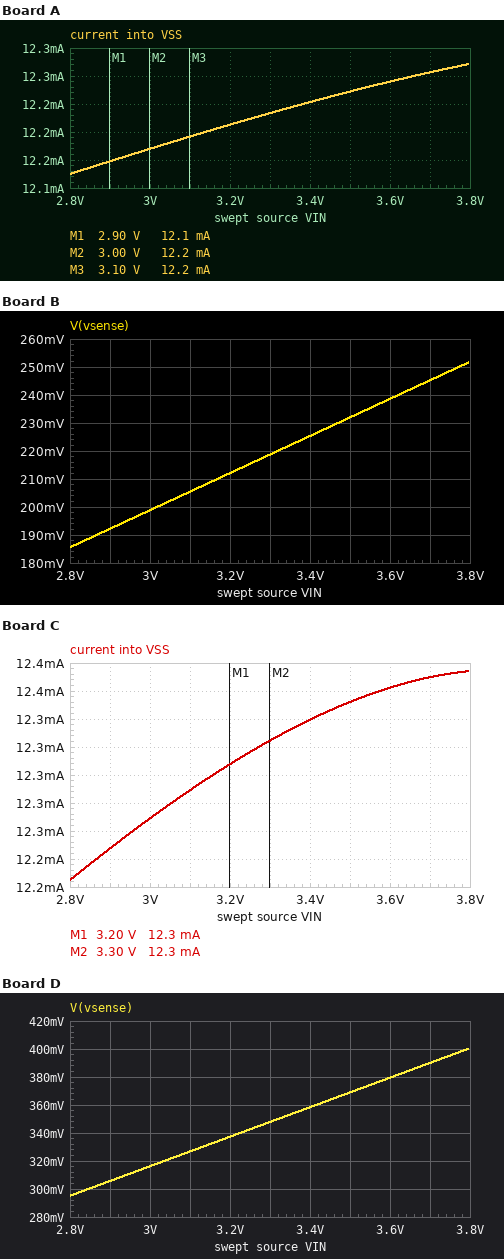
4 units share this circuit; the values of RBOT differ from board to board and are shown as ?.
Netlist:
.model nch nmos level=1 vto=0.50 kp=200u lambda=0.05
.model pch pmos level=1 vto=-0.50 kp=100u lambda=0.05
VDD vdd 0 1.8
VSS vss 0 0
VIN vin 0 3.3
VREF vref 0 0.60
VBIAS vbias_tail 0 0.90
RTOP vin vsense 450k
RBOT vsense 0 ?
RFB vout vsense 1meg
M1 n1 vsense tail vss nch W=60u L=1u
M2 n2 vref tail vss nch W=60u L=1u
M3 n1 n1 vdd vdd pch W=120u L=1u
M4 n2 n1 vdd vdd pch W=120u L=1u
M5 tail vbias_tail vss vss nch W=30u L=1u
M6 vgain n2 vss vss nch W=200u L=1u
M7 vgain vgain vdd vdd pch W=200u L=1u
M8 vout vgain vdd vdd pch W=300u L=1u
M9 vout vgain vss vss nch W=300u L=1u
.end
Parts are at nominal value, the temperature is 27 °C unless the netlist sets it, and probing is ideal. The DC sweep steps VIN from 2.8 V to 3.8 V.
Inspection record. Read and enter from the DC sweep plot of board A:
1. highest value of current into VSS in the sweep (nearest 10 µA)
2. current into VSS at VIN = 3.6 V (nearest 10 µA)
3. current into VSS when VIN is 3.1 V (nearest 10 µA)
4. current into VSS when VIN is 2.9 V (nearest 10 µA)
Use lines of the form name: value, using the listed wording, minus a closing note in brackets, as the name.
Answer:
highest value of current into VSS in the sweep: 12.32 mA
current into VSS at VIN = 3.6 V: 12.29 mA
current into VSS when VIN is 3.1 V: 12.19 mA
current into VSS when VIN is 2.9 V: 12.15 mA
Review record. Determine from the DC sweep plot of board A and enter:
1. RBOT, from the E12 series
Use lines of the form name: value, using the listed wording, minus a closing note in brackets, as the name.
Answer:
RBOT, from the E12 series: 150 kΩ
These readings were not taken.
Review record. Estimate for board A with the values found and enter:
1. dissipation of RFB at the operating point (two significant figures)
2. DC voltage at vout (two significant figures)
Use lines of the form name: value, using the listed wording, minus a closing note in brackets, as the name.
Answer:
dissipation of RFB at the operating point: 770 nW
DC voltage at vout: 1.8 V
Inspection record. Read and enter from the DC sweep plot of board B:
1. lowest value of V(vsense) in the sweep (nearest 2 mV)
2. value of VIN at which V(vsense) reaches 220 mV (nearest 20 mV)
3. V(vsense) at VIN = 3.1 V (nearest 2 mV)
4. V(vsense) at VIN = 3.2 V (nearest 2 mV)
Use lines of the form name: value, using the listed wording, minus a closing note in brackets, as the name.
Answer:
lowest value of V(vsense) in the sweep: 186 mV
value of VIN at which V(vsense) reaches 220 mV: 3.32 V
V(vsense) at VIN = 3.1 V: 206 mV
V(vsense) at VIN = 3.2 V: 212 mV
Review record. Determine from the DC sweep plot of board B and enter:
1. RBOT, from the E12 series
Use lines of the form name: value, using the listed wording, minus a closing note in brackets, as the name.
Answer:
RBOT, from the E12 series: 33 kΩ
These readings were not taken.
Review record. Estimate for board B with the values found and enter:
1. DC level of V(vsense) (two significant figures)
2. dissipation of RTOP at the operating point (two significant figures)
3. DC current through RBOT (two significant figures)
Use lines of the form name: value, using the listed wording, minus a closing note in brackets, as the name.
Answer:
DC level of V(vsense): 220 mV
dissipation of RTOP at the operating point: 21 µW
DC current through RBOT: 6.6 µA
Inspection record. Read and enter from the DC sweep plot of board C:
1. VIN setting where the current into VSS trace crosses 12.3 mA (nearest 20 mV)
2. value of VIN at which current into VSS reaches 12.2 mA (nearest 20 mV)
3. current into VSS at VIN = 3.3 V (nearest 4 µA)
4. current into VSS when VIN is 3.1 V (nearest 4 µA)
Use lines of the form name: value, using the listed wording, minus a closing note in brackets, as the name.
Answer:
VIN setting where the current into VSS trace crosses 12.3 mA: 2.96 V
value of VIN at which current into VSS reaches 12.2 mA: 2.86 V
current into VSS at VIN = 3.3 V: 12.324 mA
current into VSS when VIN is 3.1 V: 12.288 mA
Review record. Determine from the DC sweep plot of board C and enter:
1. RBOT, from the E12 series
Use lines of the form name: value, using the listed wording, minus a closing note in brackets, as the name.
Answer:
RBOT, from the E12 series: 180 kΩ
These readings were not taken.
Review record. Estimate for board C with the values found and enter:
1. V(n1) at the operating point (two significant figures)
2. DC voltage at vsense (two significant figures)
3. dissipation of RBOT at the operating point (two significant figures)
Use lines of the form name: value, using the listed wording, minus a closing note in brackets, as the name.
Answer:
V(n1) at the operating point: 1.0 V
DC voltage at vsense: 1.0 V
dissipation of RBOT at the operating point: 6.0 µW
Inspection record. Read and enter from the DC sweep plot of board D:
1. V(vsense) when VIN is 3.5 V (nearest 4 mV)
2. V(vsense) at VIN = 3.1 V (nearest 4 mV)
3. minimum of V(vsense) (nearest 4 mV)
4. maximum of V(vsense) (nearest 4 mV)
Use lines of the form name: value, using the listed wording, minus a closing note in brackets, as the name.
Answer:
V(vsense) when VIN is 3.5 V: 368 mV
V(vsense) at VIN = 3.1 V: 328 mV
minimum of V(vsense): 296 mV
maximum of V(vsense): 400 mV
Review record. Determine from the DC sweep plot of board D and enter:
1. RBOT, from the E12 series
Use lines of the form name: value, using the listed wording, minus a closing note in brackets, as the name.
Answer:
RBOT, from the E12 series: 56 kΩ
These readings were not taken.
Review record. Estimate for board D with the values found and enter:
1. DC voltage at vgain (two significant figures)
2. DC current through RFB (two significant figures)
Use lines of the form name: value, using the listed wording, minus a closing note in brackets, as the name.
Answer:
DC voltage at vgain: 1.3 V
DC current through RFB: 350 nA
